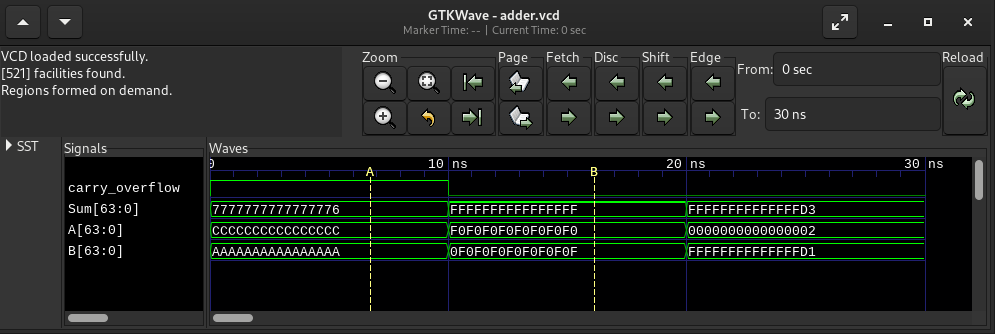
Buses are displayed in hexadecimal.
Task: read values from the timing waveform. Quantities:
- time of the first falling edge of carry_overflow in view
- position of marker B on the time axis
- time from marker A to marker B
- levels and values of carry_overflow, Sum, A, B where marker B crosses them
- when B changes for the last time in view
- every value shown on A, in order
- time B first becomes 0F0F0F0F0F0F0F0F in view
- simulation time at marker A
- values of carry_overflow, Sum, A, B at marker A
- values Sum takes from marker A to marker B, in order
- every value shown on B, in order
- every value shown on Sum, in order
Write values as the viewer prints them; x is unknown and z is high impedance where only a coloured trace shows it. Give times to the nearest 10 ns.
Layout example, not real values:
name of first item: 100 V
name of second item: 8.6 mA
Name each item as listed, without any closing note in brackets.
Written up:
time of the first falling edge of carry_overflow in view: 10 ns
position of marker B on the time axis: 20 ns
time from marker A to marker B: 10 ns
levels and values of carry_overflow, Sum, A, B where marker B crosses them: carry_overflow=0, Sum=FFFFFFFFFFFFFFFF, A=F0F0F0F0F0F0F0F0, B=0F0F0F0F0F0F0F0F
when B changes for the last time in view: 20 ns
every value shown on A, in order: CCCCCCCCCCCCCCCC, F0F0F0F0F0F0F0F0, 0000000000000002
time B first becomes 0F0F0F0F0F0F0F0F in view: 10 ns
simulation time at marker A: 10 ns
values of carry_overflow, Sum, A, B at marker A: carry_overflow=1, Sum=7777777777777776, A=CCCCCCCCCCCCCCCC, B=AAAAAAAAAAAAAAAA
values Sum takes from marker A to marker B, in order: 7777777777777776, FFFFFFFFFFFFFFFF
every value shown on B, in order: AAAAAAAAAAAAAAAA, 0F0F0F0F0F0F0F0F, FFFFFFFFFFFFFFD1
every value shown on Sum, in order: 7777777777777776, FFFFFFFFFFFFFFFF, FFFFFFFFFFFFFFD3
